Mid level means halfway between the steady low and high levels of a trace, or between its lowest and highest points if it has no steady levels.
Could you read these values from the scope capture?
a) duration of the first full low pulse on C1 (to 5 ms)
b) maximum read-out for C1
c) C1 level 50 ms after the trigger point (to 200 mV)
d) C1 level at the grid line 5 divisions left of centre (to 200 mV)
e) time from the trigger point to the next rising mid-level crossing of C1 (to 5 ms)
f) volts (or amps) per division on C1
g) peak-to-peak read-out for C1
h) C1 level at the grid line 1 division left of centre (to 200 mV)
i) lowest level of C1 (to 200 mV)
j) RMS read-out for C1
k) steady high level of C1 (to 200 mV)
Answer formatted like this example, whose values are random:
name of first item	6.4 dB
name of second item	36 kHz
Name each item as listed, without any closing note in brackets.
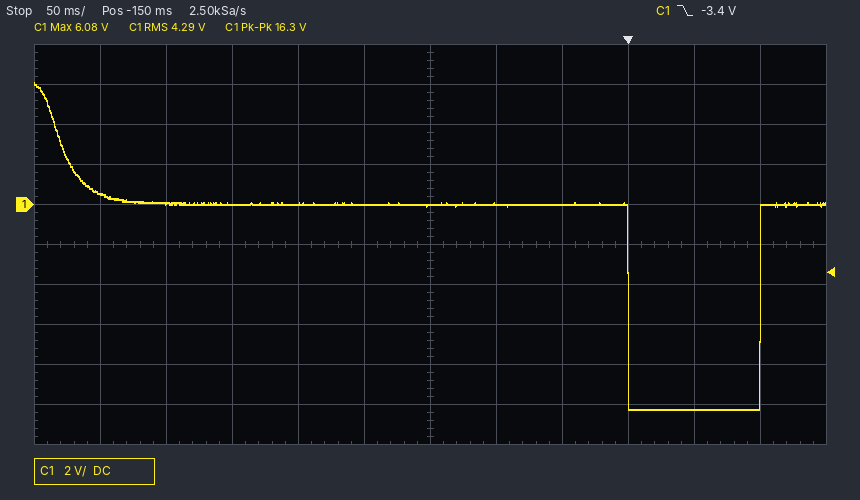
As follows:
duration of the first full low pulse on C1	100 ms
maximum read-out for C1	6.08 V
C1 level 50 ms after the trigger point	-10.2 V
C1 level at the grid line 5 divisions left of centre	600 mV
time from the trigger point to the next rising mid-level crossing of C1	100 ms
volts (or amps) per division on C1	2 V
peak-to-peak read-out for C1	16.3 V
C1 level at the grid line 1 division left of centre	0.0 V
lowest level of C1	-10.2 V
RMS read-out for C1	4.29 V
steady high level of C1	0.0 V
